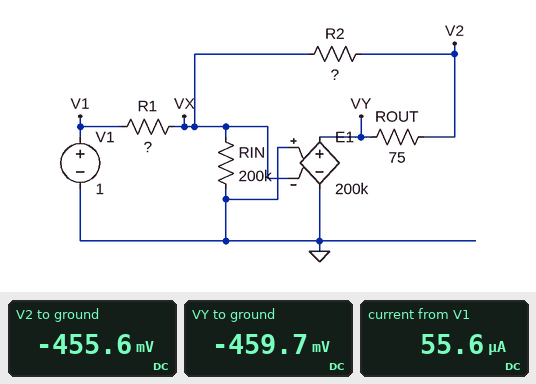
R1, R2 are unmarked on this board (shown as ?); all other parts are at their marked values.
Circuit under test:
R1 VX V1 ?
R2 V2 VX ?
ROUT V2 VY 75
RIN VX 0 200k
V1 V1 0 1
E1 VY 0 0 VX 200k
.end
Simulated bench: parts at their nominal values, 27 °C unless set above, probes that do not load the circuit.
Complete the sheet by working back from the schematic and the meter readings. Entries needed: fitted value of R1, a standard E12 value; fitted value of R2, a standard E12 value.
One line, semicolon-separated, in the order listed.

18 kΩ; 8.2 kΩ
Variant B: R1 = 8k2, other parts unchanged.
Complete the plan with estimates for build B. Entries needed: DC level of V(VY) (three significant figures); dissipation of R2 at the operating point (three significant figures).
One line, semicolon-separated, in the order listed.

-1.01 V; 122 µW
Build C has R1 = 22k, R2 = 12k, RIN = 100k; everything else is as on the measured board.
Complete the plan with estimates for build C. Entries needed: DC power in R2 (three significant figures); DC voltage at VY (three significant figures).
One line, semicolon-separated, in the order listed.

24.8 µW; -549 mV
